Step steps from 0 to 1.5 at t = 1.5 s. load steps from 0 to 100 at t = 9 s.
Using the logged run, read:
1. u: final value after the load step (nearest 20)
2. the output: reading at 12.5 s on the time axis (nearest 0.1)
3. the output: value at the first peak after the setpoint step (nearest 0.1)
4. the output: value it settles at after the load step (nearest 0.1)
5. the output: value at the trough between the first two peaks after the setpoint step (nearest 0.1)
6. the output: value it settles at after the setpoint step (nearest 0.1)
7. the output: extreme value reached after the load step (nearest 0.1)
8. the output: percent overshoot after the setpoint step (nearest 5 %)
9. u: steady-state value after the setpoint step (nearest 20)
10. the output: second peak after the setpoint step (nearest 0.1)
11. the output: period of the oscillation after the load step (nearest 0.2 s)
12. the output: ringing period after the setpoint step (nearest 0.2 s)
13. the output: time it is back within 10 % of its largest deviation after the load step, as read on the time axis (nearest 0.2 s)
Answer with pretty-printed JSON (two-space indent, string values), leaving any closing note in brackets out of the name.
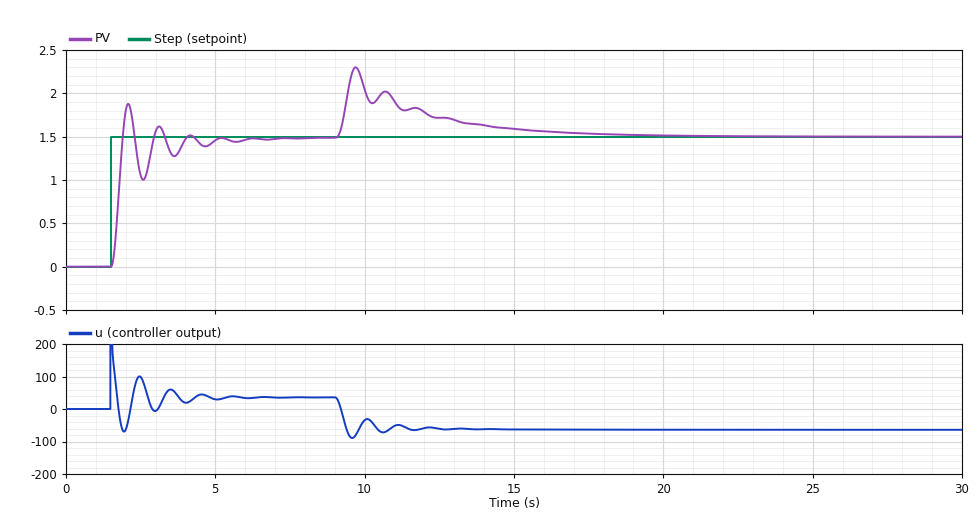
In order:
{
  "u: final value after the load step": "-60",
  "the output: reading at 12.5 s on the time axis": "1.7",
  "the output: value at the first peak after the setpoint step": "1.9",
  "the output: value it settles at after the load step": "1.5",
  "the output: value at the trough between the first two peaks after the setpoint step": "1.0",
  "the output: value it settles at after the setpoint step": "1.5",
  "the output: extreme value reached after the load step": "2.3",
  "the output: percent overshoot after the setpoint step": "25 %",
  "u: steady-state value after the setpoint step": "40",
  "the output: second peak after the setpoint step": "1.6",
  "the output: period of the oscillation after the load step": "1.0 s",
  "the output: ringing period after the setpoint step": "1.0 s",
  "the output: time it is back within 10 % of its largest deviation after the load step, as read on the time axis": "15.2 s"
}
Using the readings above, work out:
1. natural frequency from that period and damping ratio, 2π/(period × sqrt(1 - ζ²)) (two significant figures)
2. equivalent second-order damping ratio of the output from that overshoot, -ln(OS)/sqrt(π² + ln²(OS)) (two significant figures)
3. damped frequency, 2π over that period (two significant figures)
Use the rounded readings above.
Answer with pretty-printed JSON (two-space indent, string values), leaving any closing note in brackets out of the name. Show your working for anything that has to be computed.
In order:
{
  "natural frequency from that period and damping ratio, 2π/(period × sqrt(1 - ζ²))": "2π / (1 × sqrt(1 - 0.4²)) = 6.9 rad/s",
  "equivalent second-order damping ratio of the output from that overshoot, -ln(OS)/sqrt(π² + ln²(OS))": "ln(0.25) = -1.386; 1.386 / sqrt(9.870 + 1.922) = 0.40",
  "damped frequency, 2π over that period": "2π / 1 = 6.3 rad/s"
}
